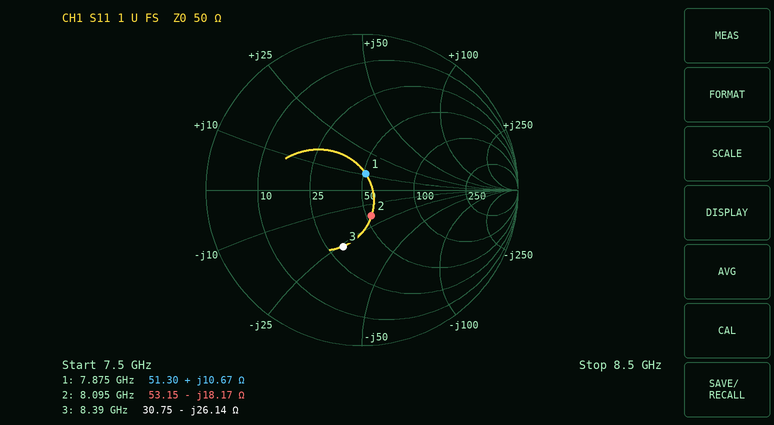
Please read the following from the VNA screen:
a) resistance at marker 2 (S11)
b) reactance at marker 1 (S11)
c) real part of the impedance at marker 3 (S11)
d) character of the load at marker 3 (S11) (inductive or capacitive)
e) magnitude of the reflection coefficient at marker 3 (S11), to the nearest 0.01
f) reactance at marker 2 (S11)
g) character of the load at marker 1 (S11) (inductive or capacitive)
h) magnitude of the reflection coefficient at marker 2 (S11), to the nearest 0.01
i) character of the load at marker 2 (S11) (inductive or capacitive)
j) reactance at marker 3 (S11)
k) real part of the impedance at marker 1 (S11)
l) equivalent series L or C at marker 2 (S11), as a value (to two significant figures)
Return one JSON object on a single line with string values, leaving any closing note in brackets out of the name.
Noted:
{"resistance at marker 2": "53.15 Ω", "reactance at marker 1": "+10.67 Ω", "real part of the impedance at marker 3": "30.75 Ω", "character of the load at marker 3 (S11)": "capacitive", "magnitude of the reflection coefficient at marker 3 (S11), to the nearest 0.01": "0.38", "reactance at marker 2": "-18.17 Ω", "character of the load at marker 1 (S11)": "inductive", "magnitude of the reflection coefficient at marker 2 (S11), to the nearest 0.01": "0.18", "character of the load at marker 2 (S11)": "capacitive", "reactance at marker 3": "-26.14 Ω", "real part of the impedance at marker 1": "51.30 Ω", "equivalent series L or C at marker 2 (S11), as a value": "1.1 pF"}
